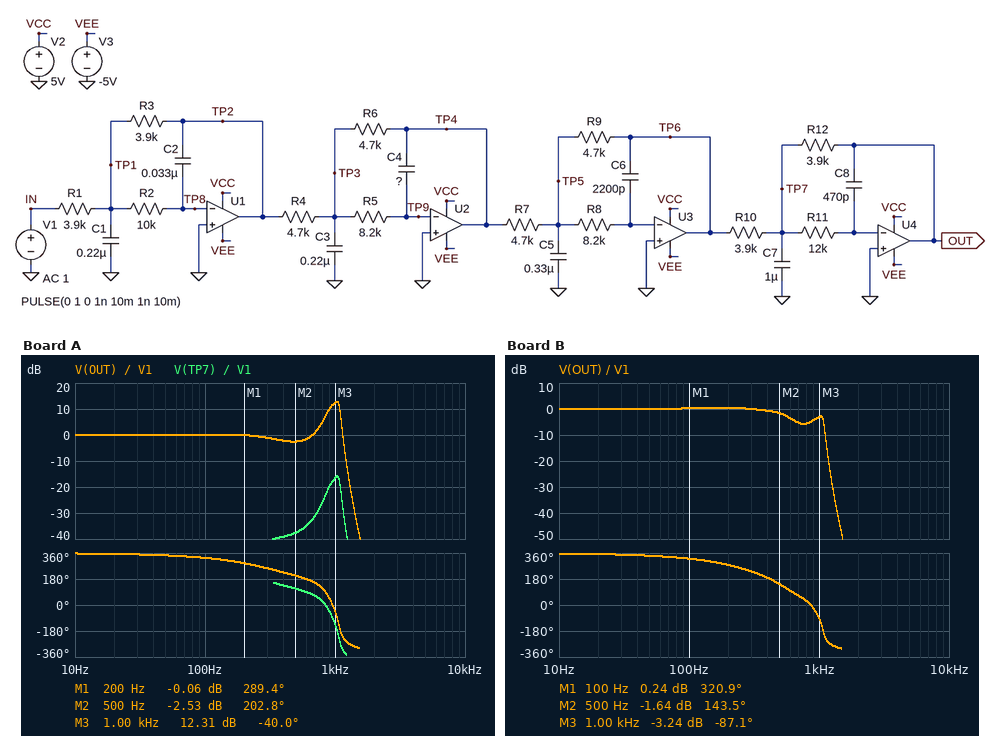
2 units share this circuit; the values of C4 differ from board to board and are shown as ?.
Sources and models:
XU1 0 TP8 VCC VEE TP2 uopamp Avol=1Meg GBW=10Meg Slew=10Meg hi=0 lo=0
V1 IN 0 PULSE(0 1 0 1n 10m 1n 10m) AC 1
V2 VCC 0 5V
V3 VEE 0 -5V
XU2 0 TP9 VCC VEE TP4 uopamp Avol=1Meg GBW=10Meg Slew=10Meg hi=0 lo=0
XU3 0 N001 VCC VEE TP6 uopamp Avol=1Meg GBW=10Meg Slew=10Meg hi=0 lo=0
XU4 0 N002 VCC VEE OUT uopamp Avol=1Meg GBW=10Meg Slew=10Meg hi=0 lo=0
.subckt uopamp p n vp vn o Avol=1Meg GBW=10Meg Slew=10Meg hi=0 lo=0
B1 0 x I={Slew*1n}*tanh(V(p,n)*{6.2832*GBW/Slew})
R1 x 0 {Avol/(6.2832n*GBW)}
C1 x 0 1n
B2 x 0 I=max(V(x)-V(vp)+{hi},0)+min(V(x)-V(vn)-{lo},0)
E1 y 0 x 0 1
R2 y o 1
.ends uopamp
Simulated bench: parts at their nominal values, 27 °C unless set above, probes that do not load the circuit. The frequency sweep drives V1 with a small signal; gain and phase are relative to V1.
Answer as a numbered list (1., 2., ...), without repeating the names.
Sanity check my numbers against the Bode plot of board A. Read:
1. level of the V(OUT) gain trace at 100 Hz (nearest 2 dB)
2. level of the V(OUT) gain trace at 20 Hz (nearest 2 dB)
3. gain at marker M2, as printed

1. 0 dB
2. 0 dB
3. -2.53 dB
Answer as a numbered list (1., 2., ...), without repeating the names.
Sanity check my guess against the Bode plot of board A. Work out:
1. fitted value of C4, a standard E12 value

1. 3.3 nF
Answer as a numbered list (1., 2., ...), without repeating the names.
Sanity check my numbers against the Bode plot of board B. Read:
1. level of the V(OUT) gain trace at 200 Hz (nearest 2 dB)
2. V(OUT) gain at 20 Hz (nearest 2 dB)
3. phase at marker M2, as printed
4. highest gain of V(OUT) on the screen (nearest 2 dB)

1. 0 dB
2. 0 dB
3. 143.5 deg
4. 0 dB
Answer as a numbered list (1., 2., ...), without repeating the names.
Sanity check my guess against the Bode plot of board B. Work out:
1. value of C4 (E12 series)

1. 10 nF
